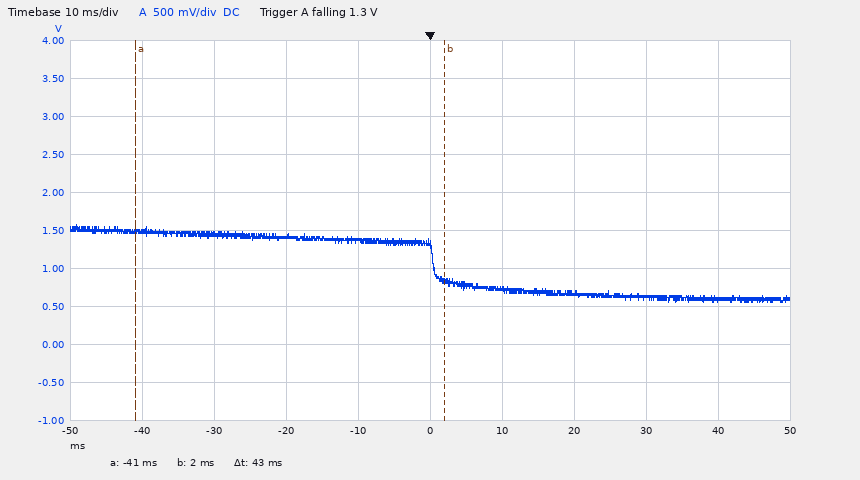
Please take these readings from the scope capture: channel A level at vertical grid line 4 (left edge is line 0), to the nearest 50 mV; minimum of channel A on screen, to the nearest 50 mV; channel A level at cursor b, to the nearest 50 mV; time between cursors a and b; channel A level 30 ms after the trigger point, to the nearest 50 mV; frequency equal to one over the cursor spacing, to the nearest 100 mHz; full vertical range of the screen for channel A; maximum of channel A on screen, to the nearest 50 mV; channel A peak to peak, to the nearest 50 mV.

1.35 V
550 mV
850 mV
43 ms
600 mV
23.3 Hz
5 V
1.60 V
1.05 V
